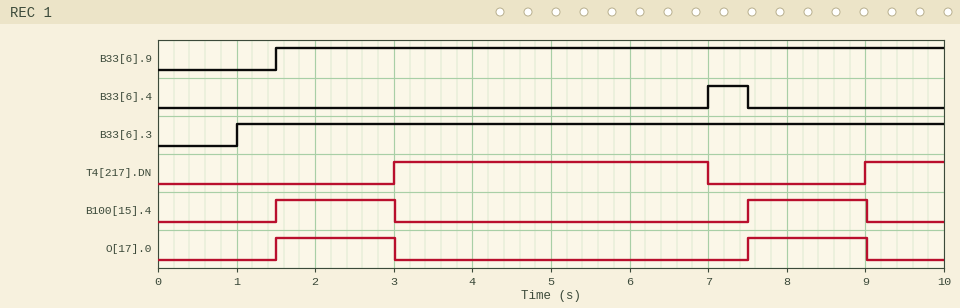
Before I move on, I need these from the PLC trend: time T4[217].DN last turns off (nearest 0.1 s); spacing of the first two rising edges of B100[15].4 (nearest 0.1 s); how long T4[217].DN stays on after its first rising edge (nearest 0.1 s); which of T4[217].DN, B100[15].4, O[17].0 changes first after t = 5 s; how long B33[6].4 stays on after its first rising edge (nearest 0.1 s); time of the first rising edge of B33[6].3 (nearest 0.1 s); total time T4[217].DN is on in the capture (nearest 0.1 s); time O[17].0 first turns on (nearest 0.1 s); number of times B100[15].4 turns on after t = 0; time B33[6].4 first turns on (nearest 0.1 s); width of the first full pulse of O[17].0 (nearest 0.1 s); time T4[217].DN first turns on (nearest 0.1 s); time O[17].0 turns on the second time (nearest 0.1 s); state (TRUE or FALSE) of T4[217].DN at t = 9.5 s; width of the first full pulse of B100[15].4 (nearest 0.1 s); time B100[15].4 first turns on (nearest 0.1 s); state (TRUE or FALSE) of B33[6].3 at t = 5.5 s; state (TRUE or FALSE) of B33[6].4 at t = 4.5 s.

7.0 s
6.0 s
4.0 s
T4[217].DN
0.5 s
1.0 s
5.0 s
1.5 s
2
7.0 s
1.5 s
3.0 s
7.5 s
TRUE
1.5 s
1.5 s
TRUE
FALSE
